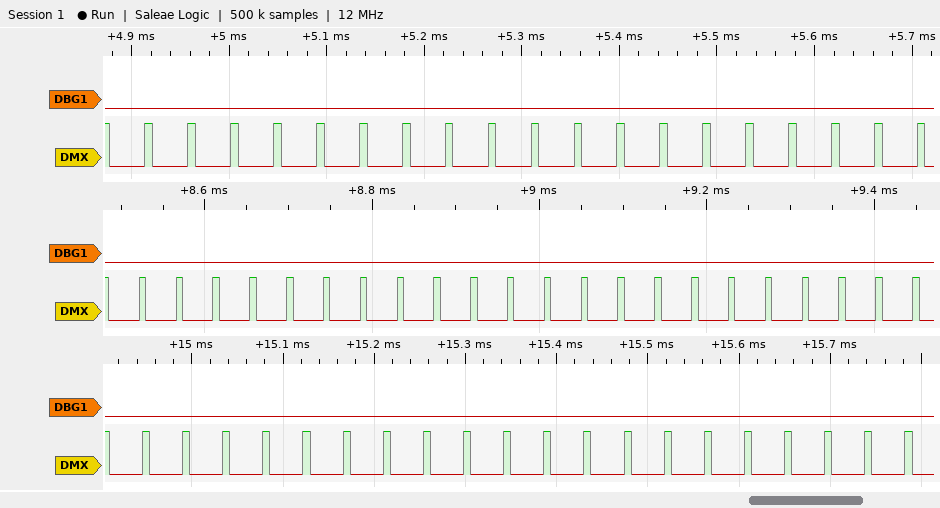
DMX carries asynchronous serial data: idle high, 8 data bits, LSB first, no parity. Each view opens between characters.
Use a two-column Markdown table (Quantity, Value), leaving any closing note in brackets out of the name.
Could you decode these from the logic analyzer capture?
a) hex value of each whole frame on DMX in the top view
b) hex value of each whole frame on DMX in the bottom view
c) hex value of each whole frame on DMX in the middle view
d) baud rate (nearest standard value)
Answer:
| Quantity | Value |
|---|---|
| hex value of each whole frame on DMX in the top view | 08, 08, 08, 08, 08, 08, 08, 08, 08 |
| hex value of each whole frame on DMX in the bottom view | 08, 08, 08, 08, 08, 08, 08, 08, 08, 08 |
| hex value of each whole frame on DMX in the middle view | 08, 08, 08, 08, 08, 08, 08, 08, 08, 08, 08 |
| baud rate | 115200 baud |
